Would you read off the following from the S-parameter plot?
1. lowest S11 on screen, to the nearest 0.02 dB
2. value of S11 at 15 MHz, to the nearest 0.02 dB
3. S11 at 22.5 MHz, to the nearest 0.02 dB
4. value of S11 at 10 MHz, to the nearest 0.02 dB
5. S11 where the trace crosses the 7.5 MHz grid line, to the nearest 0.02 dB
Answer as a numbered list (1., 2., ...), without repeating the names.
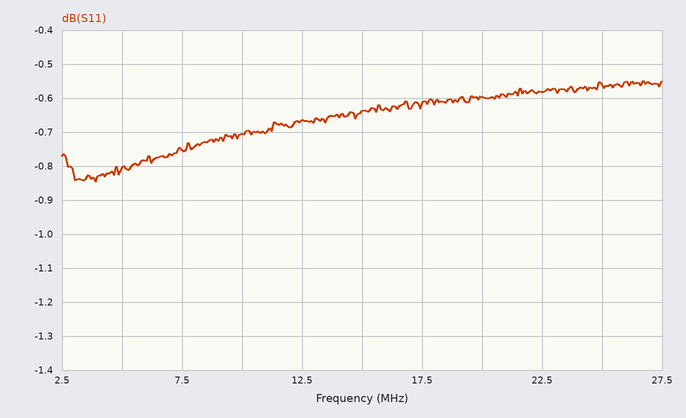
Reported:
1. -0.84 dB
2. -0.64 dB
3. -0.58 dB
4. -0.70 dB
5. -0.76 dB
